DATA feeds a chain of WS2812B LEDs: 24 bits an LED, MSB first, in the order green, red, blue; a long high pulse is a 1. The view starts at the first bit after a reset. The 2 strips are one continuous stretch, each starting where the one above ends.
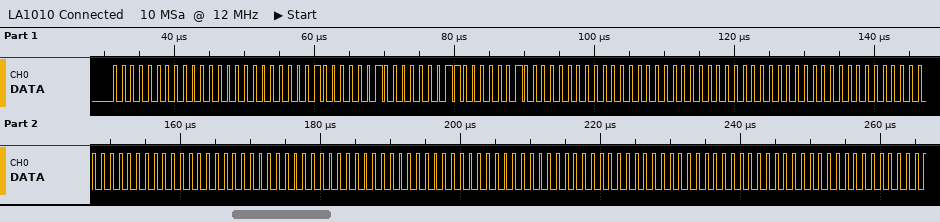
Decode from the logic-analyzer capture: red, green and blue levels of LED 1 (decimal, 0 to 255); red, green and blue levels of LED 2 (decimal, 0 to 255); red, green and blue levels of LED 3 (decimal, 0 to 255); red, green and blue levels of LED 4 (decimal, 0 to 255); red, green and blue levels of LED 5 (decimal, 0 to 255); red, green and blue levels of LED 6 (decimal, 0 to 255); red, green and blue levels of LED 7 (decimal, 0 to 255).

0, 0, 1
3, 2, 2
0, 0, 0
0, 0, 0
0, 0, 0
0, 0, 0
0, 0, 0
